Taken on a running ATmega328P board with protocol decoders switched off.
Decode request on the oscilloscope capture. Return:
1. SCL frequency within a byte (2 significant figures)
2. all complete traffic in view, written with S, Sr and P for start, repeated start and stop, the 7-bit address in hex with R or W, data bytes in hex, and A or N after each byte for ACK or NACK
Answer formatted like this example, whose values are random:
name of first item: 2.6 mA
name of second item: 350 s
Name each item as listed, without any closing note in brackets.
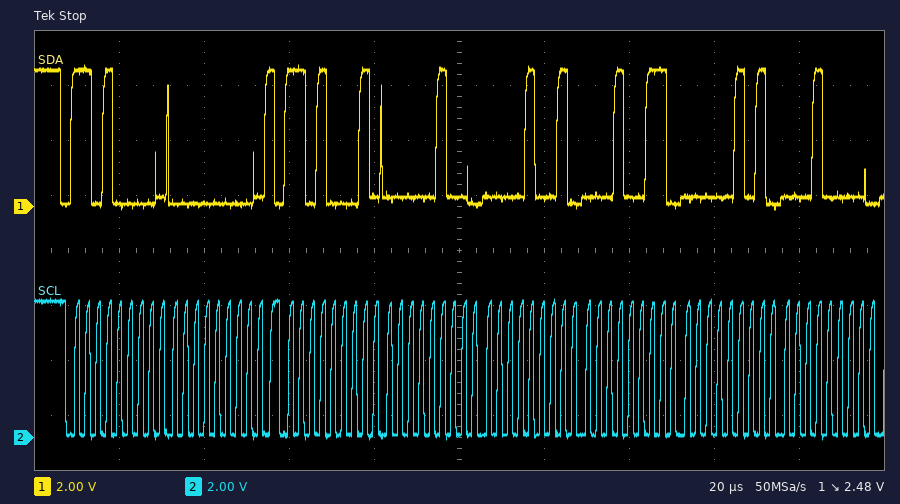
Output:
SCL frequency within a byte: 400 kHz
all complete traffic in view, written with S, Sr and P for start, repeated start and stop, the 7-bit address in hex with R or W, data bytes in hex, and A or N after each byte for ACK or NACK: S 68W A 00 A Sr 68R A 04 A 09 A 13 A 05 A 10 A
